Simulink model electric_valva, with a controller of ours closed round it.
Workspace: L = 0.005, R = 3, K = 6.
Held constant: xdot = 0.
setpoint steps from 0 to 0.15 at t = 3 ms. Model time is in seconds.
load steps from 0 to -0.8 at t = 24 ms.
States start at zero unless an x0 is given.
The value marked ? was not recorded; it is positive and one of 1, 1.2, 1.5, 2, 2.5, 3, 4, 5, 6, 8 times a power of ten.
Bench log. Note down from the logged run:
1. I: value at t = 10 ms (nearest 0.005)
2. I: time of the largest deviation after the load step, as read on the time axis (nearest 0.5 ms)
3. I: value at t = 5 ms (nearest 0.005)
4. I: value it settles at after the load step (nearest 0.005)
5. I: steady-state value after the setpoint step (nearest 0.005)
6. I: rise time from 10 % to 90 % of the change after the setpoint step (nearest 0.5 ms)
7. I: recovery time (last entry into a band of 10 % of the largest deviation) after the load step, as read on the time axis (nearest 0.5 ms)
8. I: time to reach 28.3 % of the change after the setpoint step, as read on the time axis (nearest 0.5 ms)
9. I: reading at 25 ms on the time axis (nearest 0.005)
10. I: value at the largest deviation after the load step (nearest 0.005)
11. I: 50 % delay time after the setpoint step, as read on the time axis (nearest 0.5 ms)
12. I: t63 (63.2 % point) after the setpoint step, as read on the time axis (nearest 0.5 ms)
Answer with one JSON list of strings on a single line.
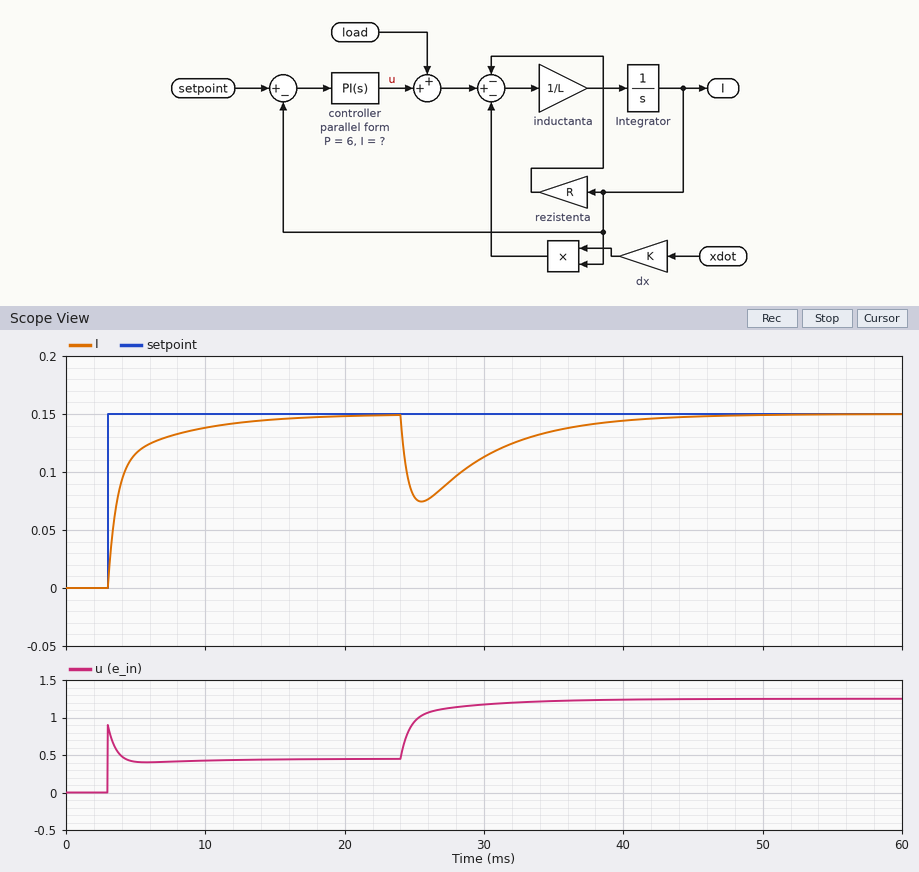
["0.140", "25.5 ms", "0.115", "0.150", "0.150", "5.5 ms", "38.5 ms", "3.5 ms", "0.080", "0.075", "3.5 ms", "4.0 ms"]
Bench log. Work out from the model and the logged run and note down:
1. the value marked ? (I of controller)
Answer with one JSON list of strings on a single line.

["1500"]
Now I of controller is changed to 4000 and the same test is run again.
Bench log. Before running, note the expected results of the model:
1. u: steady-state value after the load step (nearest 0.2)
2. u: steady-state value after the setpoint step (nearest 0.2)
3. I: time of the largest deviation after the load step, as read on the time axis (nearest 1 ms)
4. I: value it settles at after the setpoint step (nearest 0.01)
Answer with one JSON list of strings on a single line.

["1.2", "0.4", "25 ms", "0.15"]
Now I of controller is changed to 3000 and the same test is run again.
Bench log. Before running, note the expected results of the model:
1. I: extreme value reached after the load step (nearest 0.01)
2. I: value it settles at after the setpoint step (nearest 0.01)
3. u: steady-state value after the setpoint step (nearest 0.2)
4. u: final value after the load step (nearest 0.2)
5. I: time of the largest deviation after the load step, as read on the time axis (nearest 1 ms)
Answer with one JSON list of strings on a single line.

["0.08", "0.15", "0.4", "1.2", "25 ms"]
